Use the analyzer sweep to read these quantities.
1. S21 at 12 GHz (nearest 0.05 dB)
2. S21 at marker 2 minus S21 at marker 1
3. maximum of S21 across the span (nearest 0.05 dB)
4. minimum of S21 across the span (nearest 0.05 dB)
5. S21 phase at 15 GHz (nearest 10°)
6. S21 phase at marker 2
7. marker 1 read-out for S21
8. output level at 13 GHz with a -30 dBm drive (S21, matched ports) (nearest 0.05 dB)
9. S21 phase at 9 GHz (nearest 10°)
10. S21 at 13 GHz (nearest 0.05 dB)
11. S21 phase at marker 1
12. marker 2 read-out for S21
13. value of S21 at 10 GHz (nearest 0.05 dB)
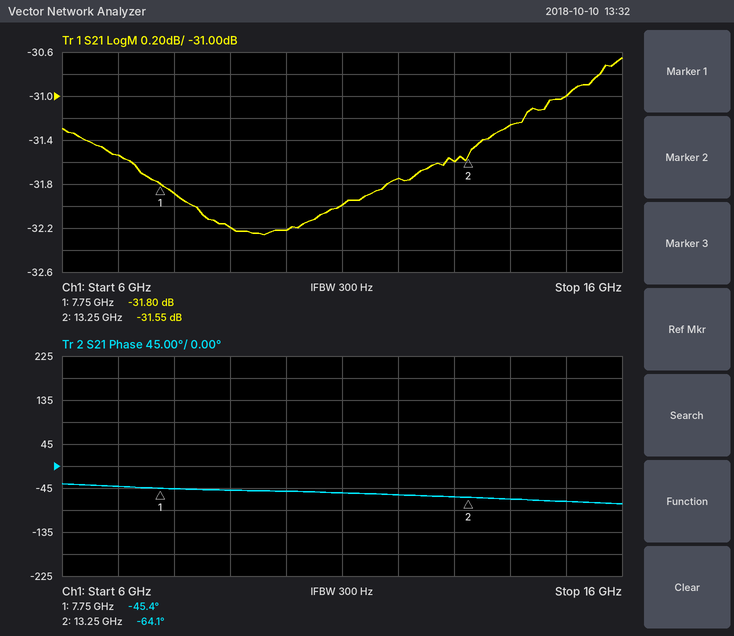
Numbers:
-31.75 dB
0.25 dB
-30.65 dB
-32.25 dB
-70°
-64.1°
-31.80 dB
-61.60 dBm
-50°
-31.60 dB
-45.4°
-31.55 dB
-32.20 dB
